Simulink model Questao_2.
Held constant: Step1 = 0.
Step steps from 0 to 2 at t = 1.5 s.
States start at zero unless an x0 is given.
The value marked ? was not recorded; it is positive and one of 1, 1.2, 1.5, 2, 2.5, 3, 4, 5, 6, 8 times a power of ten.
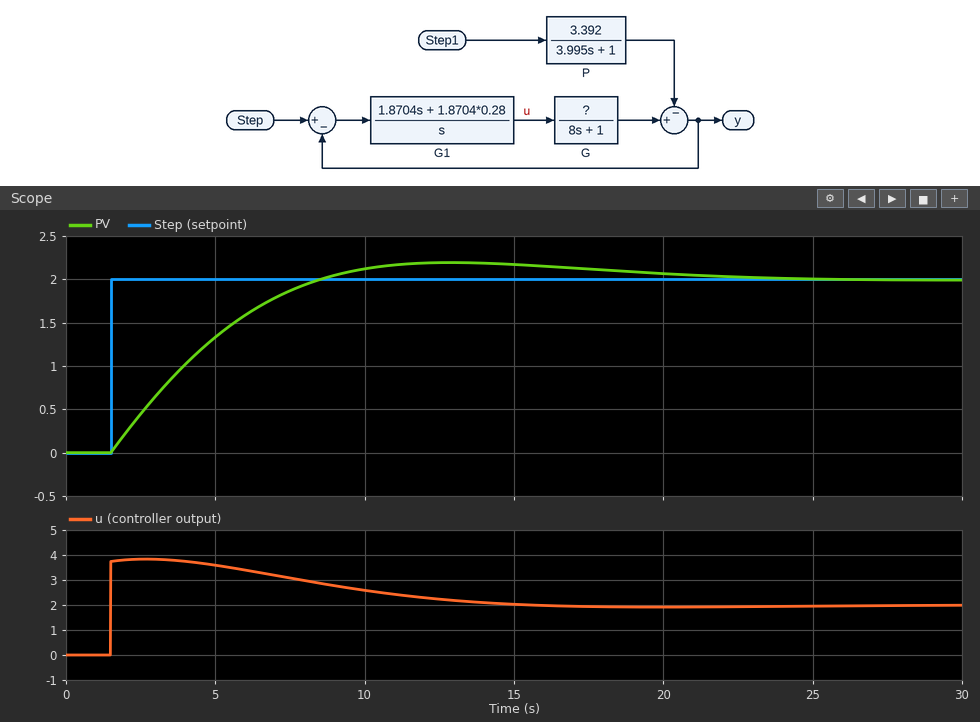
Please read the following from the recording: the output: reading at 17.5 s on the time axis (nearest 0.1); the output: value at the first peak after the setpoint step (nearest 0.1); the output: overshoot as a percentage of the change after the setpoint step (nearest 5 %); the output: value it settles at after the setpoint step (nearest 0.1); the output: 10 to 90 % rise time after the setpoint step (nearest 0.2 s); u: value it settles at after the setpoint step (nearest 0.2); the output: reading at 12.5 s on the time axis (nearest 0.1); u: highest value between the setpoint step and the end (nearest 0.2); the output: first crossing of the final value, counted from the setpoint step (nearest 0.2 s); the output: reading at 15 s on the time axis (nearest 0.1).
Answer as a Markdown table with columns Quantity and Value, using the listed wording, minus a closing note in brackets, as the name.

| Quantity | Value |
|---|---|
| the output: reading at 17.5 s on the time axis | 2.1 |
| the output: value at the first peak after the setpoint step | 2.2 |
| the output: overshoot as a percentage of the change after the setpoint step | 10 % |
| the output: value it settles at after the setpoint step | 2.0 |
| the output: 10 to 90 % rise time after the setpoint step | 5.2 s |
| u: value it settles at after the setpoint step | 2.0 |
| the output: reading at 12.5 s on the time axis | 2.2 |
| u: highest value between the setpoint step and the end | 3.8 |
| the output: first crossing of the final value, counted from the setpoint step | 7.0 s |
| the output: reading at 15 s on the time axis | 2.2 |
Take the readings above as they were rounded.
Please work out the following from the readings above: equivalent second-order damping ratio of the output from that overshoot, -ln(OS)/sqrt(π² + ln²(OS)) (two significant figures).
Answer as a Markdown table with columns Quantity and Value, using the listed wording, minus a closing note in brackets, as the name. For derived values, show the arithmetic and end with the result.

| Quantity | Value |
|---|---|
| equivalent second-order damping ratio of the output from that overshoot, -ln(OS)/sqrt(π² + ln²(OS)) | ln(0.1) = -2.303; 2.303 / sqrt(9.870 + 5.302) = 0.59 |
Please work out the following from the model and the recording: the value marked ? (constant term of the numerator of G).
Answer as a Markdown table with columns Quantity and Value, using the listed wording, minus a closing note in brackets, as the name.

| Quantity | Value |
|---|---|
| the value marked ? | 1 |
